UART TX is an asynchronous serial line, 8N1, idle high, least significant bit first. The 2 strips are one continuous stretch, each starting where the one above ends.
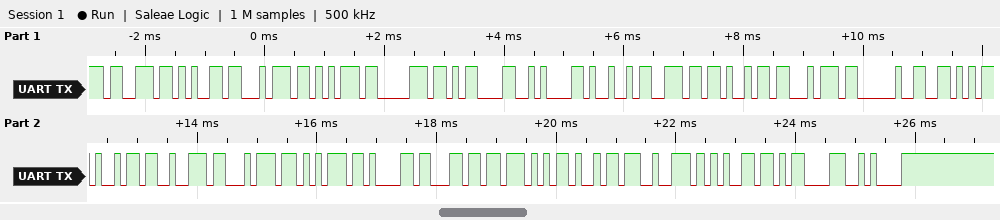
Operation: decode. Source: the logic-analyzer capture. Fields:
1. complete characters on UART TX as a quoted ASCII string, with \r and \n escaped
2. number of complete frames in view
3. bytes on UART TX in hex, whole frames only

"setup\r\nInit VirtualWire\r\n"
25
73 65 74 75 70 0D 0A 49 6E 69 74 20 56 69 72 74 75 61 6C 57 69 72 65 0D 0A
